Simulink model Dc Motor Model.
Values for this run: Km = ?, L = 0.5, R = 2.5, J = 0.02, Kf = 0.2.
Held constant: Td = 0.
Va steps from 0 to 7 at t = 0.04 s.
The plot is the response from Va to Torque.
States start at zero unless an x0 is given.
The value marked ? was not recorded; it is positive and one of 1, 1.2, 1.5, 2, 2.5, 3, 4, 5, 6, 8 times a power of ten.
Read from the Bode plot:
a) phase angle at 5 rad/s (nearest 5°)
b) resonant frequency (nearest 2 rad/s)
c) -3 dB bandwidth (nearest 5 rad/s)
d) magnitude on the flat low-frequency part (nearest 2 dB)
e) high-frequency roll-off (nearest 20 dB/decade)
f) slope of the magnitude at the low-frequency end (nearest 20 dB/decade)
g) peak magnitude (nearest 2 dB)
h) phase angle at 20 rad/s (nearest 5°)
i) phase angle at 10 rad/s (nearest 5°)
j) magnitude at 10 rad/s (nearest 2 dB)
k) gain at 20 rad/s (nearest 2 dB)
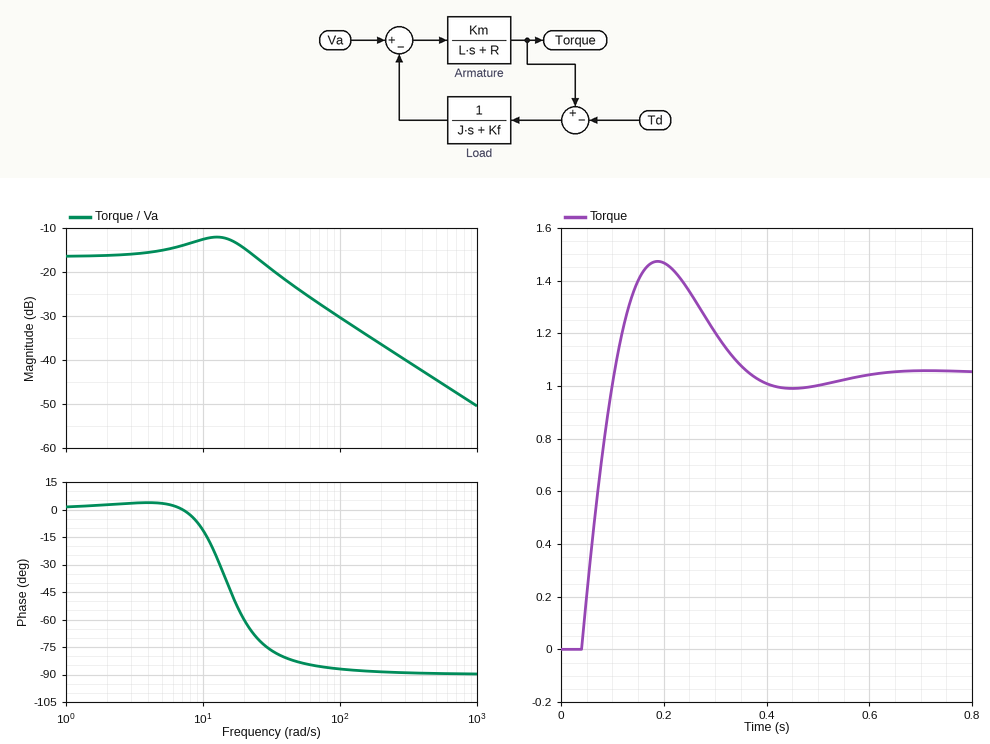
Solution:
5°
12 rad/s
30 rad/s
-16 dB
-20 dB/decade
0 dB/decade
-12 dB
-60°
-10°
-12 dB
-14 dB
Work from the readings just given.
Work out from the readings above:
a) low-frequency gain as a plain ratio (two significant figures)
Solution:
0.16
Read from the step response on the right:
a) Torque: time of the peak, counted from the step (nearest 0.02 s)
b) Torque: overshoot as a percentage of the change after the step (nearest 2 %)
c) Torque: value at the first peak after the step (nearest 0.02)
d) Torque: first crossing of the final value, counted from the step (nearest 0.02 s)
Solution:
0.14 s
40 %
1.48
0.06 s
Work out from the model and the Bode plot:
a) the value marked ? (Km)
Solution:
1.5
